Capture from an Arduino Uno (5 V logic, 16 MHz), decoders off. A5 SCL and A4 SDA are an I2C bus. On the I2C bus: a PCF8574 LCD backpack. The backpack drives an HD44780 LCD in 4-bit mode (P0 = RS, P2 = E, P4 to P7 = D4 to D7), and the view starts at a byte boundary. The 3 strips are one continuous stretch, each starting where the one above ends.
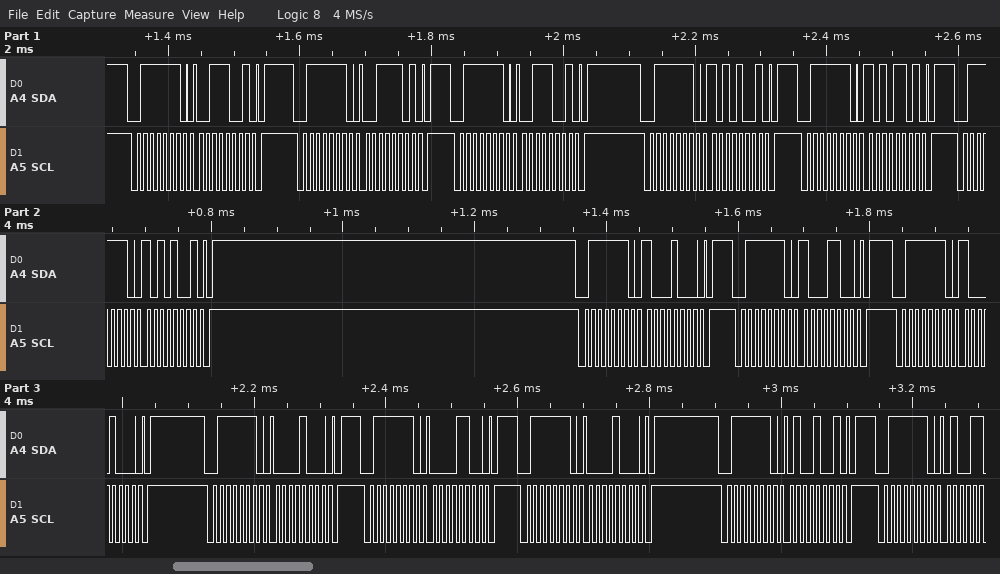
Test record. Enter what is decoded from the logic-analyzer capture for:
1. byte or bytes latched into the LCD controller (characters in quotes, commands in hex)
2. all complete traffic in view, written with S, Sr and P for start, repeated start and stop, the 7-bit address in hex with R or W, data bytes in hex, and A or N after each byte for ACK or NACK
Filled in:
':' 0x80
S 3FW A 39 A P S 3FW A 3D A P S 3FW A 39 A P S 3FW A A9 A P S 3FW A AD A P S 3FW A A9 A P S 3FW A 88 A P S 3FW A 8C A P S 3FW A 88 A P S 3FW A 08 A P S 3FW A 0C A P S 3FW A 08 A P S 3FW A 49 A P S 3FW A
